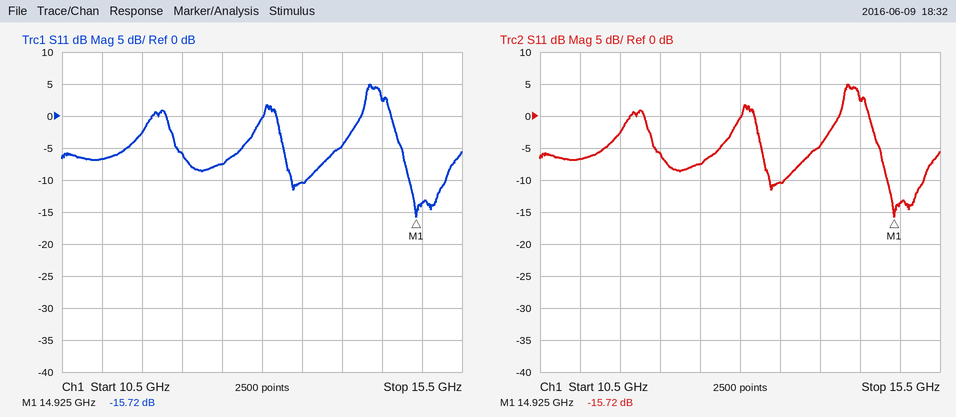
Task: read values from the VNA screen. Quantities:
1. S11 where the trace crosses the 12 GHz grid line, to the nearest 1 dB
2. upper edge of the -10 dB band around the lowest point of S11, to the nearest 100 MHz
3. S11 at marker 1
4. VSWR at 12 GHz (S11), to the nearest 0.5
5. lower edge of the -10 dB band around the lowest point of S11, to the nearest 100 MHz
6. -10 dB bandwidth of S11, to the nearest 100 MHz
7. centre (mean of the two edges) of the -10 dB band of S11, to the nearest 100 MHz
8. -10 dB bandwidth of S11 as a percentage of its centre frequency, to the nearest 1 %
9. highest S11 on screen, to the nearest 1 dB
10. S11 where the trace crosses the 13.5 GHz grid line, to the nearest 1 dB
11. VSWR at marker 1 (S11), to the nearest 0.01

-6 dB
15.3 GHz
-15.72 dB
3.0
14.8 GHz
500 MHz
15.1 GHz
3 %
5 dB
-10 dB
1.39
